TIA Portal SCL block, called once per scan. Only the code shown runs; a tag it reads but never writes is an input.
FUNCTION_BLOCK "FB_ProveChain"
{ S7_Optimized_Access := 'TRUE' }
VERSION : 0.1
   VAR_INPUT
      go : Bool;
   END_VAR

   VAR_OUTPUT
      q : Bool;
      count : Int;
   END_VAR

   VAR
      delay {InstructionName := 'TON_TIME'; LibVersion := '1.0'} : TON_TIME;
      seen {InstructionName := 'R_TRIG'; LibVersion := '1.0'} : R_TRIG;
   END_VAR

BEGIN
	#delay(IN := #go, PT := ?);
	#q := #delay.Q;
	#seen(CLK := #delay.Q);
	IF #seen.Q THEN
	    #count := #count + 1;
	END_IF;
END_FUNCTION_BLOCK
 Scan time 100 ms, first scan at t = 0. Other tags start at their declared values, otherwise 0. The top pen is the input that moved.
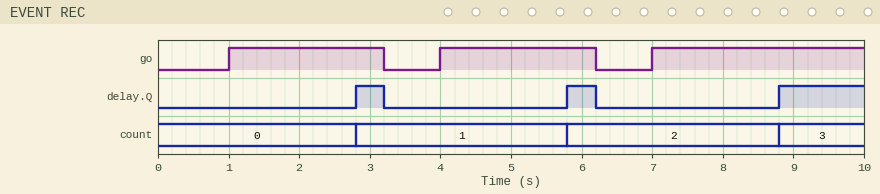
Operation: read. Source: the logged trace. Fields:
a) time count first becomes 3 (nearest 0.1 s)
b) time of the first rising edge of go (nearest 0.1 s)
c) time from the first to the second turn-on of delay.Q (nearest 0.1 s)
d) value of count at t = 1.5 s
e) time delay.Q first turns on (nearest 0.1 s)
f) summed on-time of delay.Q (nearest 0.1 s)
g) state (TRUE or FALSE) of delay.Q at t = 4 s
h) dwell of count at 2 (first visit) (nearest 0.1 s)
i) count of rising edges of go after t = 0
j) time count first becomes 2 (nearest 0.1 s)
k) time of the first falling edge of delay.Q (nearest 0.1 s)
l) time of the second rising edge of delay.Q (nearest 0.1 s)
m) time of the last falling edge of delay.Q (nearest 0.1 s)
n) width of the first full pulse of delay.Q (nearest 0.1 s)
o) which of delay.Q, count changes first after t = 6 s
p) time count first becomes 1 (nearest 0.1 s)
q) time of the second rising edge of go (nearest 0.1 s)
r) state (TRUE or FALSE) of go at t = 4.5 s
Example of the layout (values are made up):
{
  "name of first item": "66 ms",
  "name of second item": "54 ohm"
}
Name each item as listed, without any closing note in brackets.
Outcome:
{
  "time count first becomes 3": "8.8 s",
  "time of the first rising edge of go": "1.0 s",
  "time from the first to the second turn-on of delay.Q": "3.0 s",
  "value of count at t = 1.5 s": "0",
  "time delay.Q first turns on": "2.8 s",
  "summed on-time of delay.Q": "2.0 s",
  "state (TRUE or FALSE) of delay.Q at t = 4 s": "FALSE",
  "dwell of count at 2 (first visit)": "3.0 s",
  "count of rising edges of go after t = 0": "3",
  "time count first becomes 2": "5.8 s",
  "time of the first falling edge of delay.Q": "3.2 s",
  "time of the second rising edge of delay.Q": "5.8 s",
  "time of the last falling edge of delay.Q": "6.2 s",
  "width of the first full pulse of delay.Q": "0.4 s",
  "which of delay.Q, count changes first after t = 6 s": "delay.Q",
  "time count first becomes 1": "2.8 s",
  "time of the second rising edge of go": "4.0 s",
  "state (TRUE or FALSE) of go at t = 4.5 s": "TRUE"
}
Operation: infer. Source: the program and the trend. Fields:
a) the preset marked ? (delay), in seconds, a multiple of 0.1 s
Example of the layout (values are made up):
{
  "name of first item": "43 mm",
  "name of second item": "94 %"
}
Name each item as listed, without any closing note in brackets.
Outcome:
{
  "the preset marked ? (delay), in seconds, a multiple of 0.1 s": "1.8 s"
}
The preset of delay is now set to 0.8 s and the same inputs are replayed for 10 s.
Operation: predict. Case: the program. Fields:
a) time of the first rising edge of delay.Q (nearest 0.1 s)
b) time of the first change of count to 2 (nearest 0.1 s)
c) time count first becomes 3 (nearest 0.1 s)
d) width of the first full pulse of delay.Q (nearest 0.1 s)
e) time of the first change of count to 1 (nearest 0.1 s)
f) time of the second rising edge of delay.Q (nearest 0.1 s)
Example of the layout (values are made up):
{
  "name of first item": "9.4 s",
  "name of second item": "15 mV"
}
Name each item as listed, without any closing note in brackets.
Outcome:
{
  "time of the first rising edge of delay.Q": "1.8 s",
  "time of the first change of count to 2": "4.8 s",
  "time count first becomes 3": "7.8 s",
  "width of the first full pulse of delay.Q": "1.4 s",
  "time of the first change of count to 1": "1.8 s",
  "time of the second rising edge of delay.Q": "4.8 s"
}
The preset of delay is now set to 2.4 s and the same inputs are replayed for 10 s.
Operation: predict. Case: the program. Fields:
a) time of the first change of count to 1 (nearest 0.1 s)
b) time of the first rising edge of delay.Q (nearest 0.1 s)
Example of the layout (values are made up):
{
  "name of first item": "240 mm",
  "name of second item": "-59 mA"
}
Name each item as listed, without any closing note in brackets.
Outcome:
{
  "time of the first change of count to 1": "9.4 s",
  "time of the first rising edge of delay.Q": "9.4 s"
}
